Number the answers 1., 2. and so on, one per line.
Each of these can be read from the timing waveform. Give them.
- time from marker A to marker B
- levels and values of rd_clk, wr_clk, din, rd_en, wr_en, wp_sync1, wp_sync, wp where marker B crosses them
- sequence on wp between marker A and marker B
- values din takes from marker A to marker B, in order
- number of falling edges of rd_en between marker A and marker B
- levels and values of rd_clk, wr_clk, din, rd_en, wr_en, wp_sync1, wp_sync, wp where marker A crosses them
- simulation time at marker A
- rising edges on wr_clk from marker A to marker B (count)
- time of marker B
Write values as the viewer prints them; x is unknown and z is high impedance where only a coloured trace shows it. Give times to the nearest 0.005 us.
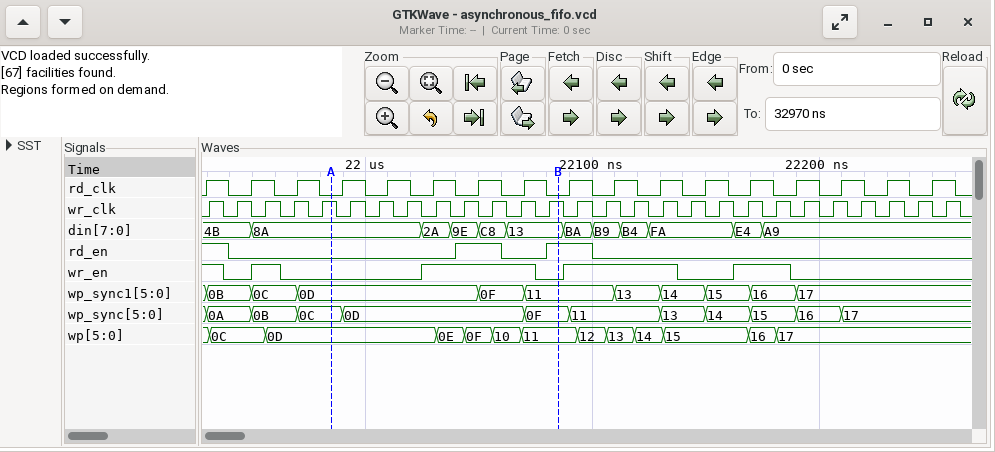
1. 0.1 us
2. rd_clk=0, wr_clk=1, din=13, rd_en=1, wr_en=0, wp_sync1=11, wp_sync=0F, wp=11
3. 0D, 0E, 0F, 10, 11
4. 8A, 2A, 9E, C8, 13
5. 1
6. rd_clk=0, wr_clk=1, din=8A, rd_en=0, wr_en=0, wp_sync1=0D, wp_sync=0C, wp=0D
7. 21.985 us
8. 8
9. 22.085 us
